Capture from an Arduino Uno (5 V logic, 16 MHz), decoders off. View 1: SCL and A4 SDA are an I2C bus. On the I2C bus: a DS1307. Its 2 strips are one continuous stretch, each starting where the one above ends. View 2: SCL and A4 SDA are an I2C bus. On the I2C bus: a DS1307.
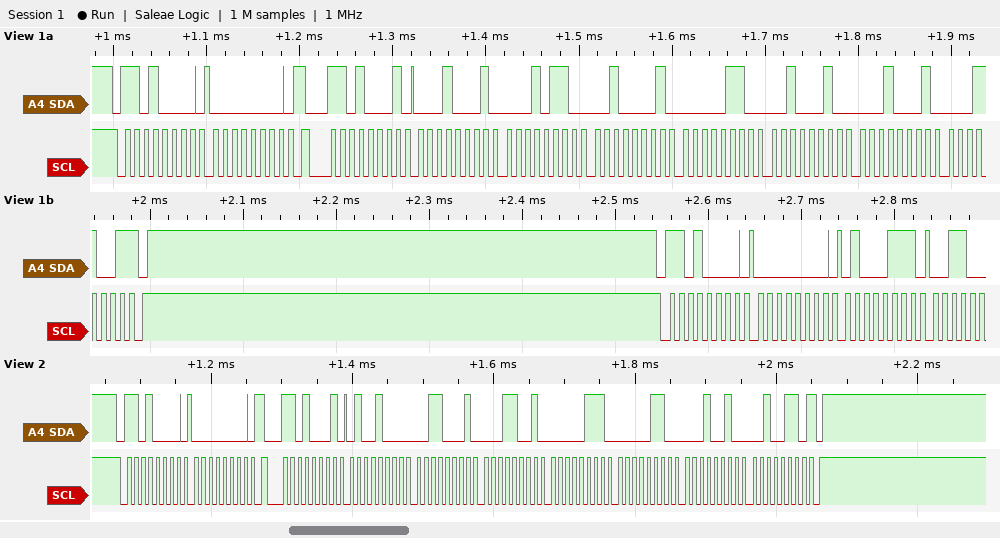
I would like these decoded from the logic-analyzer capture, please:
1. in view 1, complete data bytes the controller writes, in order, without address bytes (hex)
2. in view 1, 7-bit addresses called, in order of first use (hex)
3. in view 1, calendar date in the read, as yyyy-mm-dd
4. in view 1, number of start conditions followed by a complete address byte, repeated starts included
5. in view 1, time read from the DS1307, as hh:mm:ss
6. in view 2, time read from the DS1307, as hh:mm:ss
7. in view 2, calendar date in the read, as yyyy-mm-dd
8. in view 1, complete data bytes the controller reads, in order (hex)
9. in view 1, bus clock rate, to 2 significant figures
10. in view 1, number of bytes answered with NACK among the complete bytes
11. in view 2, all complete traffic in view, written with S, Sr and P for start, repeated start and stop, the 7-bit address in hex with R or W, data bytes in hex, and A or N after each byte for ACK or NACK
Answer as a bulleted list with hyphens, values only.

- 00 00 47
- 0x68
- 2019-11-22
- 3
- 21:16:11
- 19:31:48
- 2026-12-06
- 11 16 21 06 22 11 19
- 100 kHz
- 1
- S 68W A 00 A Sr 68R A 48 A 31 A 19 A 07 A 06 A 12 A 26 N P
